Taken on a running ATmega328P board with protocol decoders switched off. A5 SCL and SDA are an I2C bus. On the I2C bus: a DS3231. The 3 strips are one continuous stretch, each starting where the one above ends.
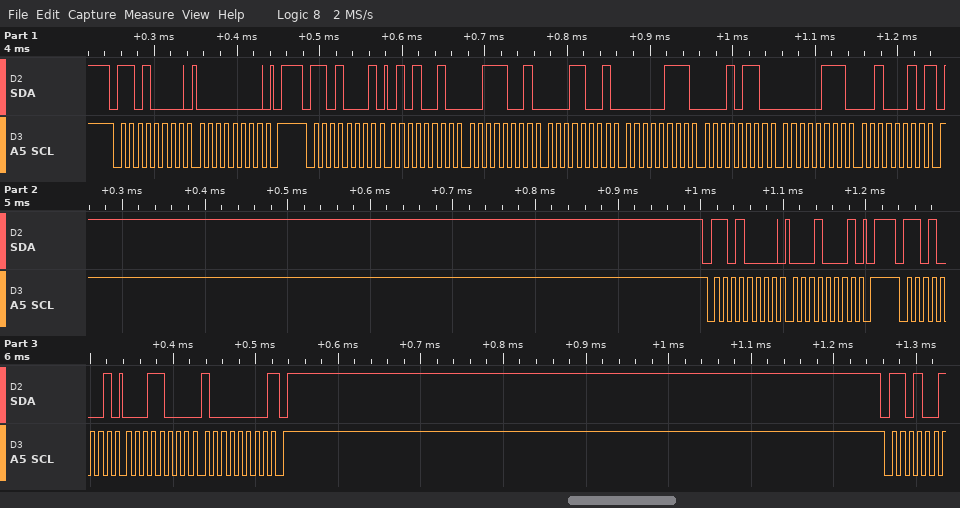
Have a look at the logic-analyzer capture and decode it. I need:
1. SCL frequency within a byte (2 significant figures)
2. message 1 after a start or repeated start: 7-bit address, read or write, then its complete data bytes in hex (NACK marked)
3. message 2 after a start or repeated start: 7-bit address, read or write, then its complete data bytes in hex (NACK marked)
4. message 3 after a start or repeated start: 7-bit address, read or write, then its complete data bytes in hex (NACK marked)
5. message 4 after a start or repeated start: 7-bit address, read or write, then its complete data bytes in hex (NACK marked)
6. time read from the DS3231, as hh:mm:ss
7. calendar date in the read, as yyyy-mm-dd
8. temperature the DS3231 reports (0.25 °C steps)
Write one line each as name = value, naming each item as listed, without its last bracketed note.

SCL frequency within a byte = 100 kHz
message 1 after a start or repeated start: 7-bit address, read or write, then its complete data bytes in hex = 0x68 write: 00
message 2 after a start or repeated start: 7-bit address, read or write, then its complete data bytes in hex = 0x68 read: 52 39 19 07 16 07 22 NACK
message 3 after a start or repeated start: 7-bit address, read or write, then its complete data bytes in hex = 0x68 write: 11
message 4 after a start or repeated start: 7-bit address, read or write, then its complete data bytes in hex = 0x68 read: 18 80 NACK
time read from the DS3231, as hh:mm:ss = 19:39:52
calendar date in the read, as yyyy-mm-dd = 2022-07-16
temperature the DS3231 reports = 24.50 °C
